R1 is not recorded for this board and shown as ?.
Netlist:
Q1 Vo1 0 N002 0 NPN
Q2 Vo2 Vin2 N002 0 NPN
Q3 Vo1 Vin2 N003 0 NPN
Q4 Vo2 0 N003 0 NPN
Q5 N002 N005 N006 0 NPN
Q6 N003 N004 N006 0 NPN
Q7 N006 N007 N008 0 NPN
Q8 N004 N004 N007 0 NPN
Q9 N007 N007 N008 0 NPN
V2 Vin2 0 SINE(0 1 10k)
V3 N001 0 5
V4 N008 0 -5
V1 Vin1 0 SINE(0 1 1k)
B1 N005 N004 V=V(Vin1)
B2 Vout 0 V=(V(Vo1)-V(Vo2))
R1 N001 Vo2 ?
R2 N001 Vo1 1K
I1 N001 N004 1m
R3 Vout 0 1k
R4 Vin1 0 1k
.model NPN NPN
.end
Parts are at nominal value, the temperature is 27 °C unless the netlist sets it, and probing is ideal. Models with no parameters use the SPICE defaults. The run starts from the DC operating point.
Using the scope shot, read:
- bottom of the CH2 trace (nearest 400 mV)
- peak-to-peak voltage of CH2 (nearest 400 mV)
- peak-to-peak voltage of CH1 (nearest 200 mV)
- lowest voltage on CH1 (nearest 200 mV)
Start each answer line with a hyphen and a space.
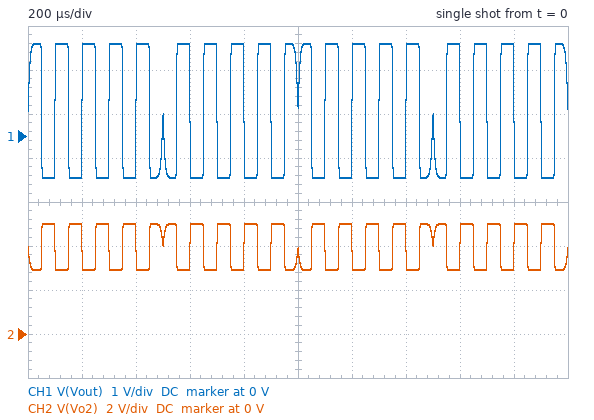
- 2.8 V
- 2.0 V
- 3.0 V
- -1.0 V
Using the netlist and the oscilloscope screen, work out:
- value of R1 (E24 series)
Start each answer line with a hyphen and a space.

- 2.2 kΩ
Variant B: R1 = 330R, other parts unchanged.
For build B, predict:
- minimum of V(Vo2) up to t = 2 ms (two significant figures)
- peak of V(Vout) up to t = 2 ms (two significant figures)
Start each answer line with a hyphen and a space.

- 4.7 V
- 310 mV
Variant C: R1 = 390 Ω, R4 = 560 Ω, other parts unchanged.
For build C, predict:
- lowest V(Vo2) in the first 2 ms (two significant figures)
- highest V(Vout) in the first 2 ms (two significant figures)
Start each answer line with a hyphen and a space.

- 4.6 V
- 370 mV
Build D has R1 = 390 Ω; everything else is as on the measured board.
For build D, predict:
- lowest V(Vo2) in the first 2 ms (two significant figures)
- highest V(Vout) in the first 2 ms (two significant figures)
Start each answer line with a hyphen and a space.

- 4.6 V
- 370 mV
